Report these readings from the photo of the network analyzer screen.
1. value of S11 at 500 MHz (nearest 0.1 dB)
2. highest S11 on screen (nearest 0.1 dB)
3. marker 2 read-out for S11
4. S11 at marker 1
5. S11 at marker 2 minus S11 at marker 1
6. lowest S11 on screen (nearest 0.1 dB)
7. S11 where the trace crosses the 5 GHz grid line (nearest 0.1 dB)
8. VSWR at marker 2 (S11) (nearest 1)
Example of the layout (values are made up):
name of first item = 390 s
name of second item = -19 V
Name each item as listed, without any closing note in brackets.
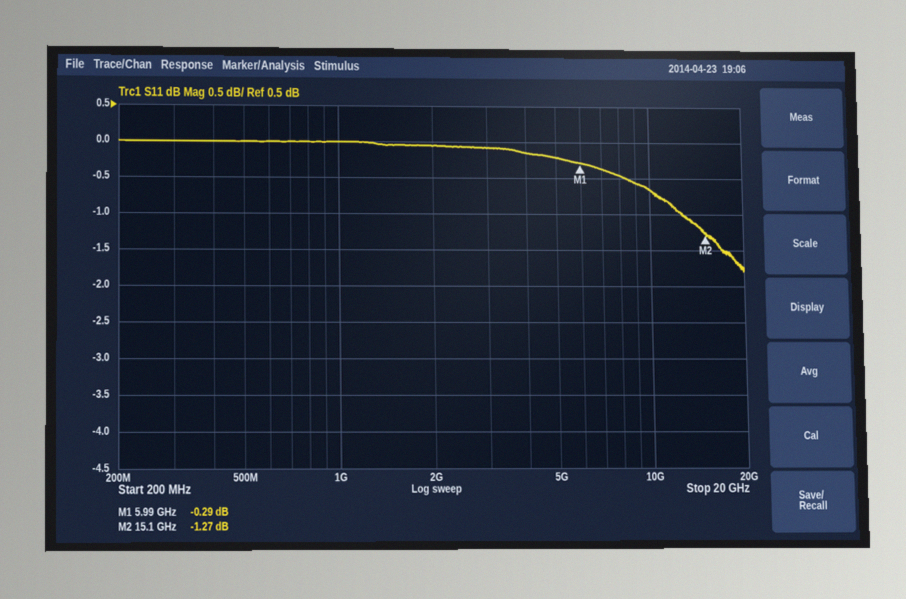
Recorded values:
value of S11 at 500 MHz = 0.0 dB
highest S11 on screen = 0.0 dB
marker 2 read-out for S11 = -1.27 dB
S11 at marker 1 = -0.29 dB
S11 at marker 2 minus S11 at marker 1 = -0.98 dB
lowest S11 on screen = -1.8 dB
S11 where the trace crosses the 5 GHz grid line = -0.2 dB
VSWR at marker 2 (S11) = 14
